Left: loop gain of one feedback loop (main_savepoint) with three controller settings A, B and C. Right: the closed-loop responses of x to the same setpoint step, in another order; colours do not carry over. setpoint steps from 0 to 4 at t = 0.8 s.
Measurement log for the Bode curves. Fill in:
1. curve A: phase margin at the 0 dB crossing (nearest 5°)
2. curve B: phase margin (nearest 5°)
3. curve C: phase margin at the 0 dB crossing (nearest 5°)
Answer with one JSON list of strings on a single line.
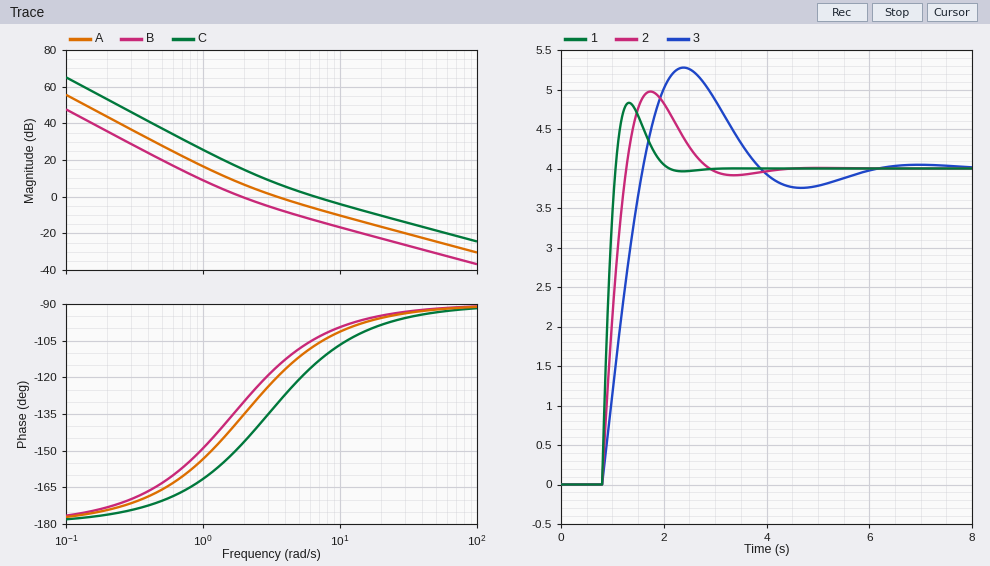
["60°", "50°", "65°"]
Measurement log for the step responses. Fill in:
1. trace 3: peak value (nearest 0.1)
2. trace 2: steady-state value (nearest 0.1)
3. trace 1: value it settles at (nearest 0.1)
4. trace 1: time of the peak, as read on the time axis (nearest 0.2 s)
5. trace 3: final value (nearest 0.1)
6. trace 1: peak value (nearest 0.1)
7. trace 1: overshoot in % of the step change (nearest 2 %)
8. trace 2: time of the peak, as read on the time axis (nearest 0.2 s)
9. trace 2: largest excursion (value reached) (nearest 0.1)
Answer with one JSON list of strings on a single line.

["5.3", "4.0", "4.0", "1.4 s", "4.0", "4.8", "20 %", "1.8 s", "5.0"]
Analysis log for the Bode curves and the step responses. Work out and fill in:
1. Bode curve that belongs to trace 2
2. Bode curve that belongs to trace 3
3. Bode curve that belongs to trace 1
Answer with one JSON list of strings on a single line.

["A", "B", "C"]
